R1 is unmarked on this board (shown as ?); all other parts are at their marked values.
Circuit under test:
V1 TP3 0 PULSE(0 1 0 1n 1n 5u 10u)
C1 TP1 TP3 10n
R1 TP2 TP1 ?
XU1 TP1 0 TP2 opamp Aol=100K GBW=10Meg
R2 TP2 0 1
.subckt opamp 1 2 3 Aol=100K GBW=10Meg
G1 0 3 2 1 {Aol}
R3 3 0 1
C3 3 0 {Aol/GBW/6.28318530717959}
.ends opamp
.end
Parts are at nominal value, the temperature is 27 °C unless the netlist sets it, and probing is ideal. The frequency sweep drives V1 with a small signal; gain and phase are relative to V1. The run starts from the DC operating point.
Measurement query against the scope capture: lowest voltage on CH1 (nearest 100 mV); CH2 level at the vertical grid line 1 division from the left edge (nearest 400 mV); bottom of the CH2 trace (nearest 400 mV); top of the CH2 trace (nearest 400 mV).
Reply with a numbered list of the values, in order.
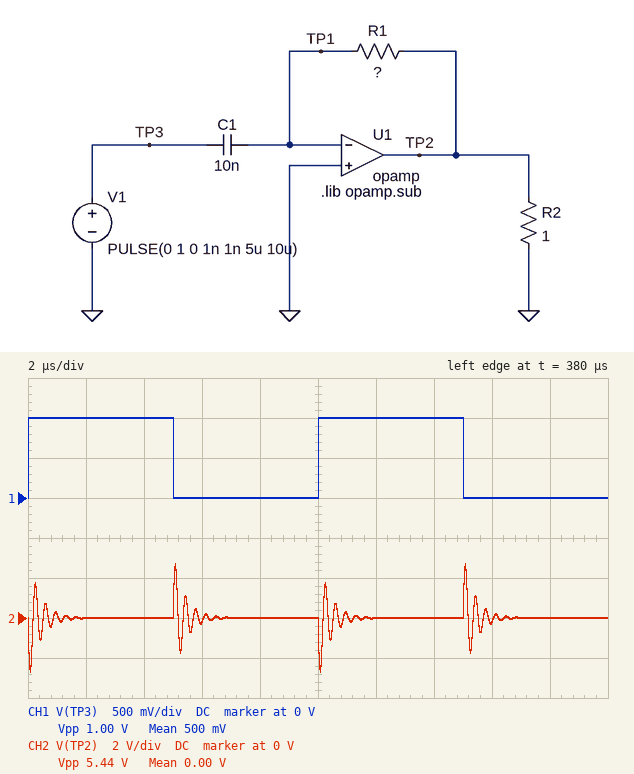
1. 0 V
2. 0 V
3. -2.8 V
4. 2.8 V
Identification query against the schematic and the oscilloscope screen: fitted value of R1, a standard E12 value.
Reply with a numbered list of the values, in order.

1. 18 Ω
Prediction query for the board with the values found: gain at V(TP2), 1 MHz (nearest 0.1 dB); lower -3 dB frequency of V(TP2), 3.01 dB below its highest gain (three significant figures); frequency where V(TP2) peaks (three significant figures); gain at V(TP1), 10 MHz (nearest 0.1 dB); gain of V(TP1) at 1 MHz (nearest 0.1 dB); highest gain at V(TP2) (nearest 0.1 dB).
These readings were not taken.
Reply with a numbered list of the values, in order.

1. 2.1 dB
2. 2.56 MHz
3. 2.97 MHz
4. 0.8 dB
5. -17.9 dB
6. 21.1 dB
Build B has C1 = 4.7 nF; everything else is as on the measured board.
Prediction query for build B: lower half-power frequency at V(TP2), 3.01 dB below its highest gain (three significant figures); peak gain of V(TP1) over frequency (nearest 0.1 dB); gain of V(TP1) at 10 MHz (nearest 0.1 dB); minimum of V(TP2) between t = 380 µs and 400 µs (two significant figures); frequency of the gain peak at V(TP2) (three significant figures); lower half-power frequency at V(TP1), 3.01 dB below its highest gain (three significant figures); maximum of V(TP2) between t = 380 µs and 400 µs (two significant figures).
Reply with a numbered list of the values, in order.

1. 3.50 MHz
2. 7.5 dB
3. 1.6 dB
4. -1.7 V
5. 4.34 MHz
6. 3.76 MHz
7. 1.7 V
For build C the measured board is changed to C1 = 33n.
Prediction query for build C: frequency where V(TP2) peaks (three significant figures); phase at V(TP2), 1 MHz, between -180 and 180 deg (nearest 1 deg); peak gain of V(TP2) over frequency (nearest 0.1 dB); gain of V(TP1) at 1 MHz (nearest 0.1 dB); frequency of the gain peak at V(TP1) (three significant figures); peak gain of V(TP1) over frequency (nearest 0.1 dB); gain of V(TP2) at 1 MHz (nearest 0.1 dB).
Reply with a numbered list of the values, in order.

1. 1.64 MHz
2. -99 deg
3. 31.4 dB
4. -4.6 dB
5. 1.65 MHz
6. 15.7 dB
7. 15.4 dB
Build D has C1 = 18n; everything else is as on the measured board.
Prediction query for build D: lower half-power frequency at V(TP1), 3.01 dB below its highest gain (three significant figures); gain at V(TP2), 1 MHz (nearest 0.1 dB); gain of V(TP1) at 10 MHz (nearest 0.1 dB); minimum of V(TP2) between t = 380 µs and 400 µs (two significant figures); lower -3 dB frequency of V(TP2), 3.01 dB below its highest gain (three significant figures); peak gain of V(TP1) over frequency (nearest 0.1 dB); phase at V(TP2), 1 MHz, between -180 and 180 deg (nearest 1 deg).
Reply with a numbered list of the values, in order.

1. 2.03 MHz
2. 8.1 dB
3. 0.4 dB
4. -3.8 V
5. 1.98 MHz
6. 13.1 dB
7. -97 deg
